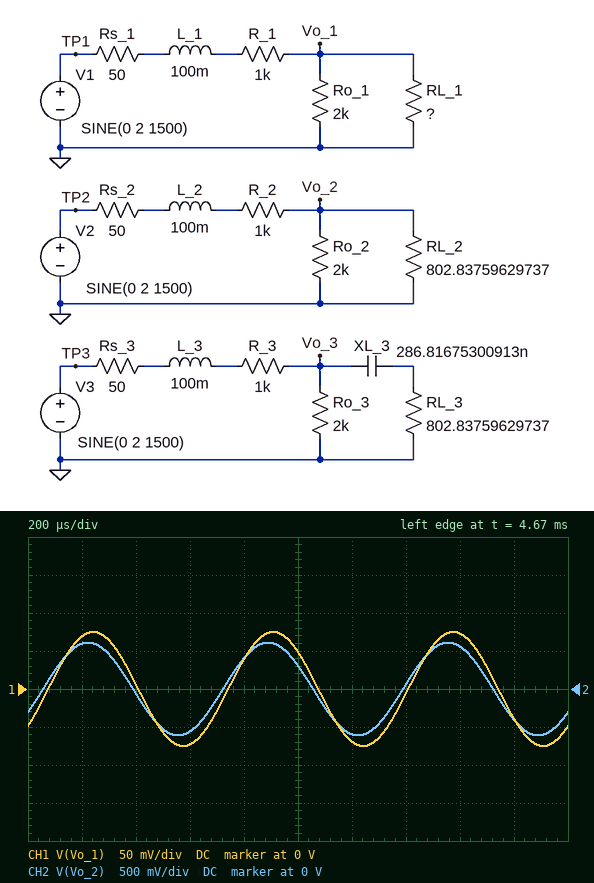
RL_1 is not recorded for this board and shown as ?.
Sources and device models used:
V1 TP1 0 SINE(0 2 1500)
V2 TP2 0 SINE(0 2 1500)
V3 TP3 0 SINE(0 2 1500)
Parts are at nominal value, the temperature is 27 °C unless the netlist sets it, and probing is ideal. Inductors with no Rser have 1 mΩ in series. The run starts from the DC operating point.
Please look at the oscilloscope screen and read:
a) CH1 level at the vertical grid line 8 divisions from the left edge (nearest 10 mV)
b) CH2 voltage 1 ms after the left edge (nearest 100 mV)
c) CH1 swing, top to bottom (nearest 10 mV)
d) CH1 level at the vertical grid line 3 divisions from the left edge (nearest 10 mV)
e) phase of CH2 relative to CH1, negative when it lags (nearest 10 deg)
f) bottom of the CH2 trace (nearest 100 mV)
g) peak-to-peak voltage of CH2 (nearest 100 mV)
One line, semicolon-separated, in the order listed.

70 mV; 300 mV; 150 mV; -70 mV; 10 deg; -600 mV; 1.2 V
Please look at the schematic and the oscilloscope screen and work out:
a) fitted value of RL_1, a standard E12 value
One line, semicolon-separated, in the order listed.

56 Ω
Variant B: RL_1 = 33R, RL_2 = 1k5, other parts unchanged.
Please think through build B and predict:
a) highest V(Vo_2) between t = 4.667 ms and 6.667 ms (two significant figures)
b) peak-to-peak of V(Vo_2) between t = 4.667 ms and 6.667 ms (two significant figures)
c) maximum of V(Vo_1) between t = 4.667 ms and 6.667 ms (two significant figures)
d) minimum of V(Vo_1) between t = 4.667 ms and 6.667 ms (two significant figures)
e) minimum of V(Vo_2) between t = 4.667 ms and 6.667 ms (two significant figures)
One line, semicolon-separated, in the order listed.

810 mV; 1.6 V; 45 mV; -45 mV; -810 mV
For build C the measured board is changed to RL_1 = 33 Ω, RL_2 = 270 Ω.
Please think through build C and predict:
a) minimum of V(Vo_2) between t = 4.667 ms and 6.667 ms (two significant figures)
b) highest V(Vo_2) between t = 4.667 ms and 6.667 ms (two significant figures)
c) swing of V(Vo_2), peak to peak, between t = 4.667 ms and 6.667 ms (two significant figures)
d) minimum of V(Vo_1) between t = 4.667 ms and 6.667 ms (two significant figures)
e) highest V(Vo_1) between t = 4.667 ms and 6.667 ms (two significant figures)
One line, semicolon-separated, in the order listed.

-300 mV; 300 mV; 600 mV; -45 mV; 45 mV
